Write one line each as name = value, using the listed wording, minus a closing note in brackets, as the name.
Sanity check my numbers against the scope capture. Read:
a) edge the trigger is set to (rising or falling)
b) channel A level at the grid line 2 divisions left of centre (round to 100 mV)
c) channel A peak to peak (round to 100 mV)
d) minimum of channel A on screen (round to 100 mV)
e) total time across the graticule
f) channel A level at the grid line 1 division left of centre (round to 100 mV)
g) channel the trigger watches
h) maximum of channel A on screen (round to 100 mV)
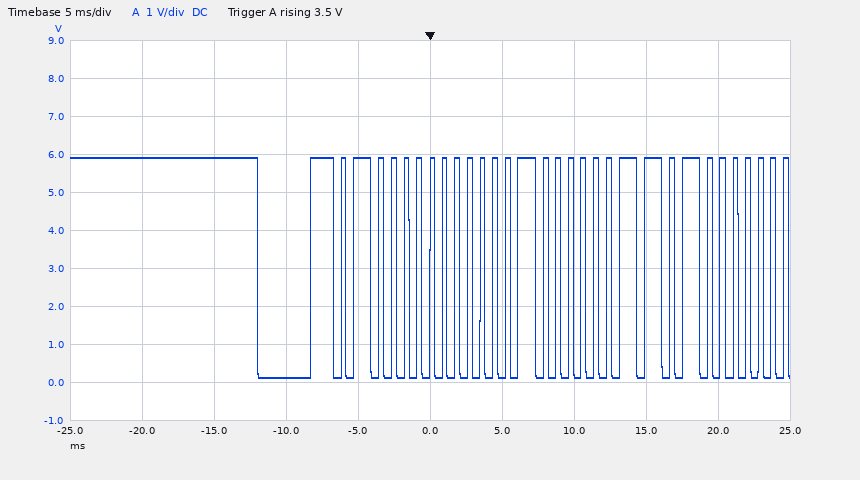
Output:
edge the trigger is set to = rising
channel A level at the grid line 2 divisions left of centre = 100 mV
channel A peak to peak = 5.8 V
minimum of channel A on screen = 100 mV
total time across the graticule = 50 ms
channel A level at the grid line 1 division left of centre = 5.9 V
channel the trigger watches = channel A
maximum of channel A on screen = 5.9 V
